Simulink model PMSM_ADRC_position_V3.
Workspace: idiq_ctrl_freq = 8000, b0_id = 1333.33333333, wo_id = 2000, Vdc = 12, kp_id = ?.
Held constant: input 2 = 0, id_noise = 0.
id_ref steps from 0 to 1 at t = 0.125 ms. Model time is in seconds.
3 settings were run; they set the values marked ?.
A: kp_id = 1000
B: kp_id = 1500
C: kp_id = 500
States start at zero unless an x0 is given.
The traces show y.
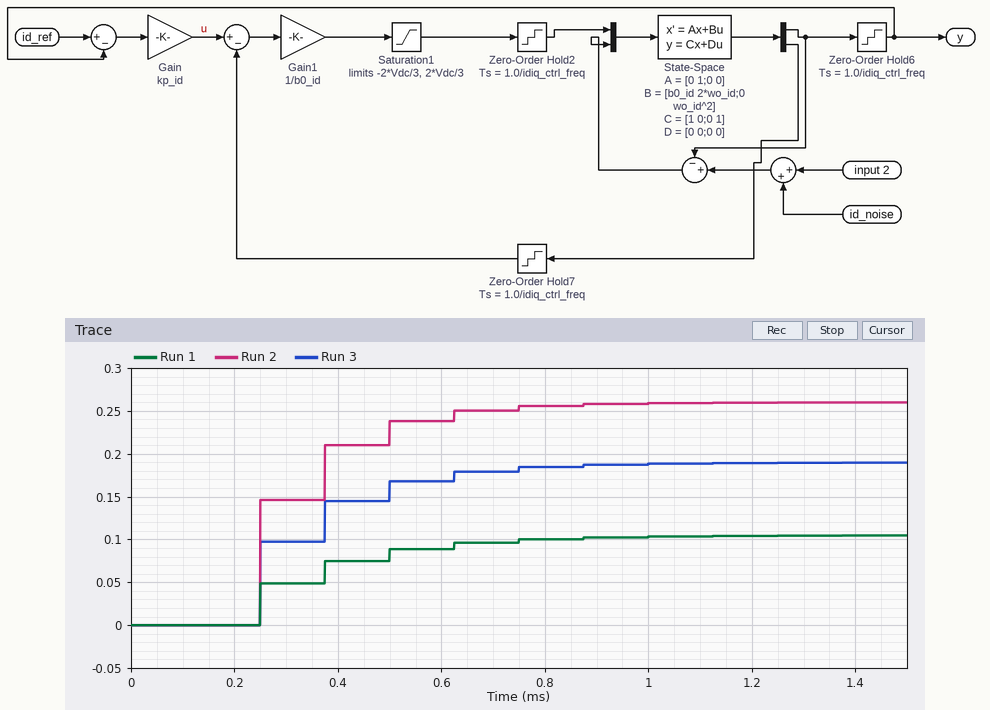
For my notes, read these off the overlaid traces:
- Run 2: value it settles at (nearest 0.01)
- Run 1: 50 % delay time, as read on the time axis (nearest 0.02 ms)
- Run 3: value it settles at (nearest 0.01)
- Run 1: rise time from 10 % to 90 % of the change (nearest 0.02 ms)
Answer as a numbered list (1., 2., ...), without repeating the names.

1. 0.26
2. 0.38 ms
3. 0.19
4. 0.38 ms
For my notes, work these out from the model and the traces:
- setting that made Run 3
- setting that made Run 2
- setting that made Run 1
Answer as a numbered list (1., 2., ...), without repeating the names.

1. A
2. B
3. C
